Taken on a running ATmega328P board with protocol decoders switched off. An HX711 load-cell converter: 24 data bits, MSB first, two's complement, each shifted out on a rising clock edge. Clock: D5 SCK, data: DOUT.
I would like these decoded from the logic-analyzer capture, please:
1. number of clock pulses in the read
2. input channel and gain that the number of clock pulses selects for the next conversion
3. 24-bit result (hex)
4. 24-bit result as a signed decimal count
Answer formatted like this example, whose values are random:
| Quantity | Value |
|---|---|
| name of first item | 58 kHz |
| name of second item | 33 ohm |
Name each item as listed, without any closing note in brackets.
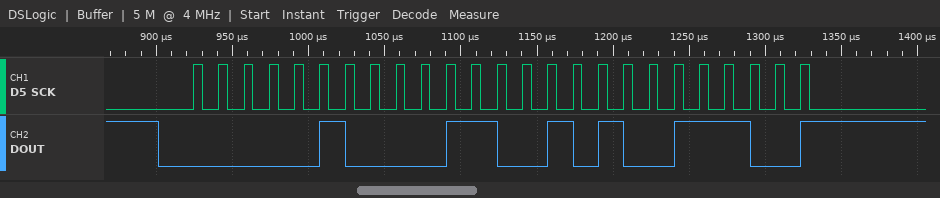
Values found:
| Quantity | Value |
|---|---|
| number of clock pulses in the read | 25 |
| input channel and gain that the number of clock pulses selects for the next conversion | channel A, gain 128 |
| 24-bit result | 0x04329C |
| 24-bit result as a signed decimal count | 275100 |
